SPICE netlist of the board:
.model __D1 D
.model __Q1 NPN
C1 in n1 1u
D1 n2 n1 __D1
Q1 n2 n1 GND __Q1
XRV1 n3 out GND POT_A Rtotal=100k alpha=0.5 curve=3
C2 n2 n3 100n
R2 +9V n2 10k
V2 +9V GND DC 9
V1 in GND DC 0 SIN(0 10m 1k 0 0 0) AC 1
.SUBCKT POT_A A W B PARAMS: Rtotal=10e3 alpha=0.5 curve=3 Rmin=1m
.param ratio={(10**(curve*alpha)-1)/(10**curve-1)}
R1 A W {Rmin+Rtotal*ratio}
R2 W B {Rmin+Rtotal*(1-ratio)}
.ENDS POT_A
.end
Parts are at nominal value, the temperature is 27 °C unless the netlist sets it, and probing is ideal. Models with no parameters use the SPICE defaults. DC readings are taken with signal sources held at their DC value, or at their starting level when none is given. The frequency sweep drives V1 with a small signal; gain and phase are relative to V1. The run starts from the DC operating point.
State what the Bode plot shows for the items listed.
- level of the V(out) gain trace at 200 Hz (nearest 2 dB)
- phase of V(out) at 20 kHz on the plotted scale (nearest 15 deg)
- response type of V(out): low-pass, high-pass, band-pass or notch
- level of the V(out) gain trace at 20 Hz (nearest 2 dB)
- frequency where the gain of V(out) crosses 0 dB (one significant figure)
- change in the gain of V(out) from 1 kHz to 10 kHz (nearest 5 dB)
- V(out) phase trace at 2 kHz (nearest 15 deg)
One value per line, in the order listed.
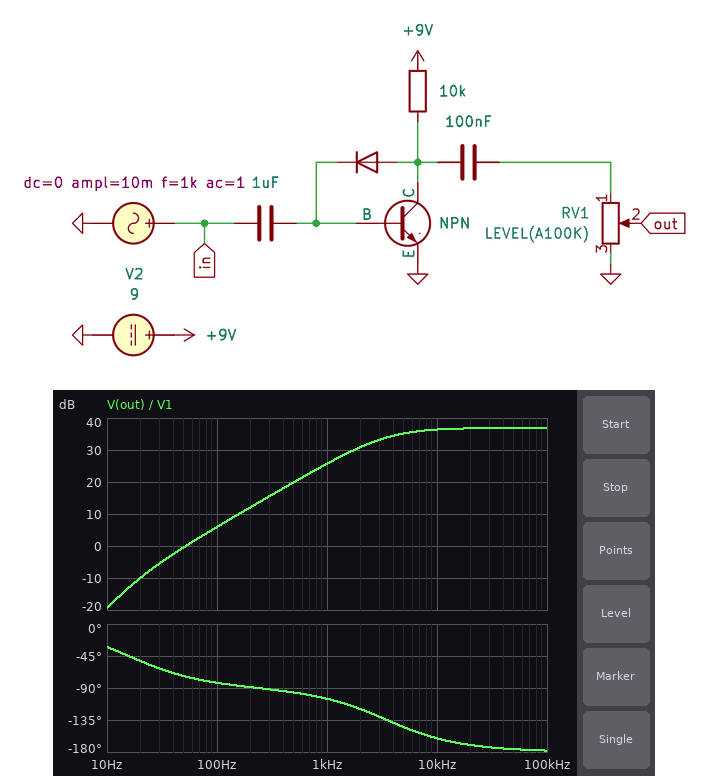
12 dB
-165 deg
high-pass
-10 dB
50 Hz
10 dB
-120 deg
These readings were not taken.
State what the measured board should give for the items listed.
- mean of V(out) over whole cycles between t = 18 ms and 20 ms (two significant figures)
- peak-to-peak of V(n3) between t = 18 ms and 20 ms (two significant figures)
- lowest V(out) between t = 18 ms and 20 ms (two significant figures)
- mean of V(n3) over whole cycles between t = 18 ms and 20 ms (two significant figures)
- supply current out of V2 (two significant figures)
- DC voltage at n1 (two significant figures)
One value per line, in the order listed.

-77 mV
1.3 V
-750 mV
-79 mV
770 µA
770 mV
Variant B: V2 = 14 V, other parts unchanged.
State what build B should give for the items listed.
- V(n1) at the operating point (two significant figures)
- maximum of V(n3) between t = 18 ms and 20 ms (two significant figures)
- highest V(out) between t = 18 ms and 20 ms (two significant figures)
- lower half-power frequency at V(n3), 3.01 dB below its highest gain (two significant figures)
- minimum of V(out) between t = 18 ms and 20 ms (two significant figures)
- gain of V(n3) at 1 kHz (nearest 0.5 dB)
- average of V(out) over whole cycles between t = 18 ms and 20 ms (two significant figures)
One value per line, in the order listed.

780 mV
490 mV
470 mV
6.4 kHz
-780 mV
22.0 dB
-74 mV
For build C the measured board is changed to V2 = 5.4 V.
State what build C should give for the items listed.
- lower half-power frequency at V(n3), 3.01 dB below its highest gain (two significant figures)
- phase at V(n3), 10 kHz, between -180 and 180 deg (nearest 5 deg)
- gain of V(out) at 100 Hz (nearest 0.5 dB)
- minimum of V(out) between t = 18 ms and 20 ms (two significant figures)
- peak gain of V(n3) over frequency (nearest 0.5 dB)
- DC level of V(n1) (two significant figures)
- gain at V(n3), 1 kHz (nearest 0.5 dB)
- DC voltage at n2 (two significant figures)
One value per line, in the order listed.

1.5 kHz
-170 deg
11.5 dB
-730 mV
35.5 dB
750 mV
30.0 dB
1.3 V
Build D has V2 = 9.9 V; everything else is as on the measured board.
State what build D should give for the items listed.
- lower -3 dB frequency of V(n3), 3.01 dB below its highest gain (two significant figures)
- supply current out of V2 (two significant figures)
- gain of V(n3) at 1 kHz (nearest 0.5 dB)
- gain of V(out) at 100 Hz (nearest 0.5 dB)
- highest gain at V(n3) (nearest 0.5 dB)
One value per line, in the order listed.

4.0 kHz
860 µA
25.0 dB
5.0 dB
37.5 dB
